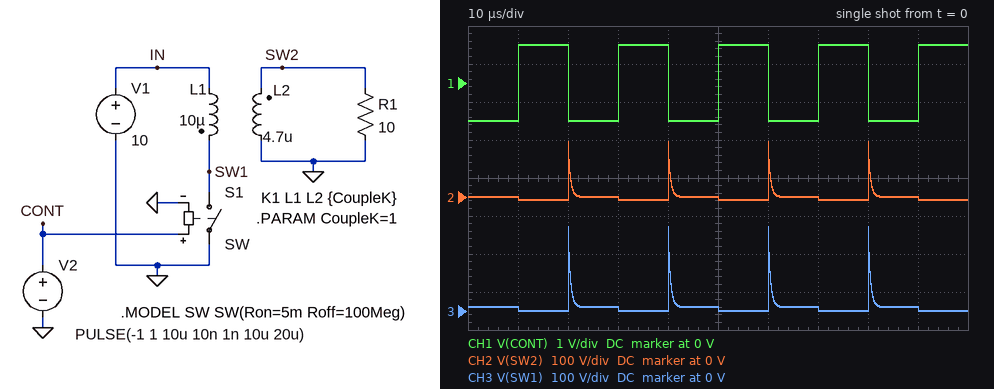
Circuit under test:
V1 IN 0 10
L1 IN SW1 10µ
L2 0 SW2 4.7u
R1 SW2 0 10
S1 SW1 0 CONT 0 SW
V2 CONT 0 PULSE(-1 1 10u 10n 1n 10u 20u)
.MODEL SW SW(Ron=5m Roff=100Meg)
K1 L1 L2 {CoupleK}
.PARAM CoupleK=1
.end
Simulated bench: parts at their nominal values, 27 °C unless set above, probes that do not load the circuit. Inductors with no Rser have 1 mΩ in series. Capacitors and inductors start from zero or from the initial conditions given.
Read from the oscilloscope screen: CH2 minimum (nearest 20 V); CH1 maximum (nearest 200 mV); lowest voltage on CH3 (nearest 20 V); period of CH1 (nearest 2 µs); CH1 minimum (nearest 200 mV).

0 V
1.0 V
0 V
20 µs
-1.0 V
